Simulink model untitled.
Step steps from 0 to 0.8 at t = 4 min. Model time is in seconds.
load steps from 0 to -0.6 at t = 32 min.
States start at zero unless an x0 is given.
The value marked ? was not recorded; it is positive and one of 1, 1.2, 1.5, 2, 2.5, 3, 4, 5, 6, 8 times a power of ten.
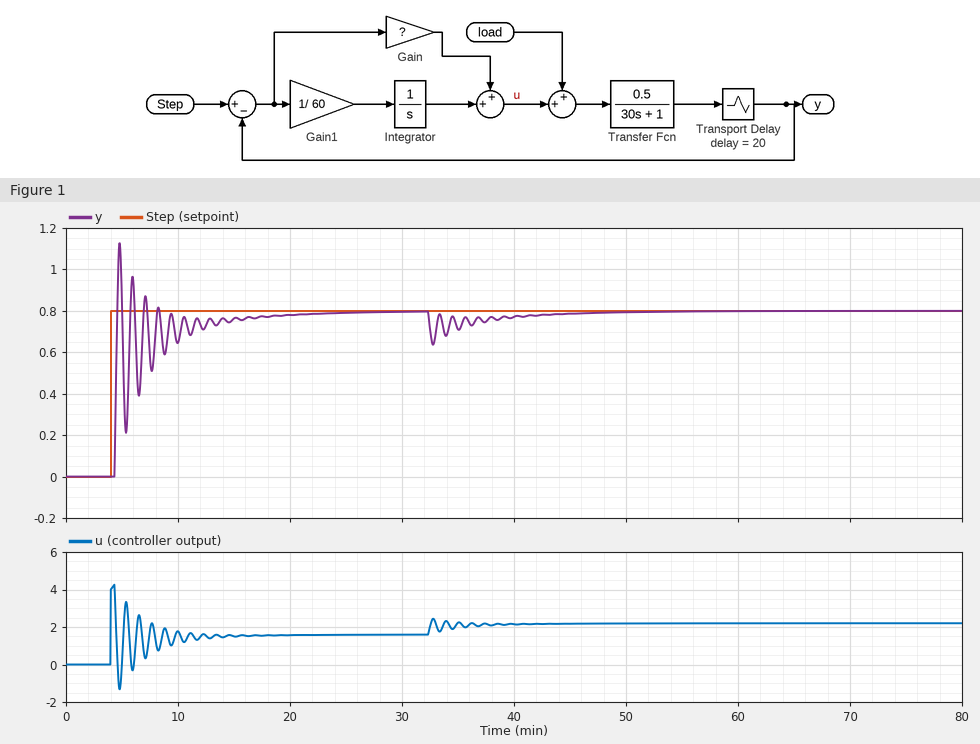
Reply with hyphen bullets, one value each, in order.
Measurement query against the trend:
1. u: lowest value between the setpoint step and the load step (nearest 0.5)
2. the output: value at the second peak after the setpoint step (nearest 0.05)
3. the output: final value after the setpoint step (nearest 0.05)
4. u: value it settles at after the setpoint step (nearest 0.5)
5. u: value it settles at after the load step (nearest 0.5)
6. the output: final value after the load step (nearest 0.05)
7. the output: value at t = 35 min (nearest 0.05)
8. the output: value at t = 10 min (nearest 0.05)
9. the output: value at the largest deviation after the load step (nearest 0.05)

- -1.5
- 0.95
- 0.80
- 1.5
- 2.0
- 0.80
- 0.70
- 0.65
- 0.65
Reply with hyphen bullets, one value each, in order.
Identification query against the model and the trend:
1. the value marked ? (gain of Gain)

- 5
